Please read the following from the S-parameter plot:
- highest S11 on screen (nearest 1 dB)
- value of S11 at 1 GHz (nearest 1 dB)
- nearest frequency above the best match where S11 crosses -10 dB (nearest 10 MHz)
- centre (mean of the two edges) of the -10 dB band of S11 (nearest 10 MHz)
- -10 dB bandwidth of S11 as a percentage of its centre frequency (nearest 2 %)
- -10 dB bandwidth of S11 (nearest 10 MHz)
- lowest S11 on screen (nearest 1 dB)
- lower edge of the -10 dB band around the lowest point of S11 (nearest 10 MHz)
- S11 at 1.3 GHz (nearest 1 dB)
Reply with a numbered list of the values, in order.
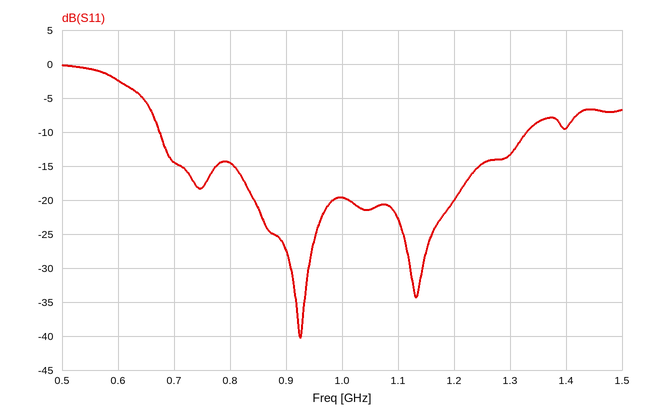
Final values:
1. 0 dB
2. -20 dB
3. 1.33 GHz
4. 1.00 GHz
5. 66 %
6. 660 MHz
7. -40 dB
8. 670 MHz
9. -13 dB
